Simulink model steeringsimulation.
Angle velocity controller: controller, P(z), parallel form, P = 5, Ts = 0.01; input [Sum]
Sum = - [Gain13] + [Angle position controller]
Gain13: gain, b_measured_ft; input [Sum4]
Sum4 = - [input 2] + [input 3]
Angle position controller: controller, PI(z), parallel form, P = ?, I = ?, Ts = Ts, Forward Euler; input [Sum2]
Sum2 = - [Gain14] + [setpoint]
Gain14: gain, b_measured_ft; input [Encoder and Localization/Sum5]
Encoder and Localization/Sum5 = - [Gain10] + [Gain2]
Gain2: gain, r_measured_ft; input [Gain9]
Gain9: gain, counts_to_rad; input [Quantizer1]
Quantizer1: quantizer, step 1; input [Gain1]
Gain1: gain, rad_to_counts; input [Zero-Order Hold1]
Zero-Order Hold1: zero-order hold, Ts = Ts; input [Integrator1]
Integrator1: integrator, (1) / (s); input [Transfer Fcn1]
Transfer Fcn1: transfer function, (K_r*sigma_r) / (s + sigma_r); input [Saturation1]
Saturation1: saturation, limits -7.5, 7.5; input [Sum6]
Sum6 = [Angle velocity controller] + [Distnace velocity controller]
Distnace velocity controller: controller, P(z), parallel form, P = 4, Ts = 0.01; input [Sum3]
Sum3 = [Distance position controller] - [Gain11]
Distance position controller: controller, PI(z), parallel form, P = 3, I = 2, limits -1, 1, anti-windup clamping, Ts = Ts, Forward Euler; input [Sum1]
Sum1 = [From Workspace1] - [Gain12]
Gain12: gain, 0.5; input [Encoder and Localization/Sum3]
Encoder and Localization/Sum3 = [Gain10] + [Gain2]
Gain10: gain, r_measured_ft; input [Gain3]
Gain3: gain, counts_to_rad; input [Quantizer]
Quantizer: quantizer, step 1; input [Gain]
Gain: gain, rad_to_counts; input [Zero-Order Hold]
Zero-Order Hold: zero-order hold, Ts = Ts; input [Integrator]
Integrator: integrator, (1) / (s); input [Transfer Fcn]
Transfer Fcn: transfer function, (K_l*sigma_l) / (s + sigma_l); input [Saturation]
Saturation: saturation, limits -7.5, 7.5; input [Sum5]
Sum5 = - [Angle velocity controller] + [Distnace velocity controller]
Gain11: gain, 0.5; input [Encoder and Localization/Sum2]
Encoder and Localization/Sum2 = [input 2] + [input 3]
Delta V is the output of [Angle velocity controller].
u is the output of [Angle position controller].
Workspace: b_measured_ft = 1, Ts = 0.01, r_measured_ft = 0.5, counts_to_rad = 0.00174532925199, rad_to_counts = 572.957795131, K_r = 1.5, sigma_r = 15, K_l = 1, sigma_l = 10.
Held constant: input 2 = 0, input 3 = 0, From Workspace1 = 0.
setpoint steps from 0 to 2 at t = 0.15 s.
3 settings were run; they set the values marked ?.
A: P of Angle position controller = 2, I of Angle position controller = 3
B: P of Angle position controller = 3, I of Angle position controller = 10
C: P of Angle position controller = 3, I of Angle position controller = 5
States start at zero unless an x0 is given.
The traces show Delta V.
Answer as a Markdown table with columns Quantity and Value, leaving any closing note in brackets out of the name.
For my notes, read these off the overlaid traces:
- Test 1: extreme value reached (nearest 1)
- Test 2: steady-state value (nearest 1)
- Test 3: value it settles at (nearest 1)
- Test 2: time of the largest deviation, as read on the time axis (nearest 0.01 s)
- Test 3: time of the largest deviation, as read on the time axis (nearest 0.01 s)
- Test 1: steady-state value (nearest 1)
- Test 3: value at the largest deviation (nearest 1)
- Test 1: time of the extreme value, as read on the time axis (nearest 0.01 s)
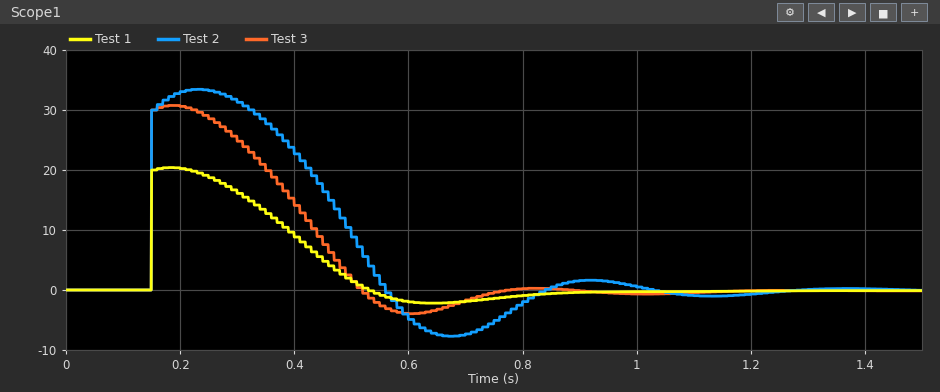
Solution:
| Quantity | Value |
|---|---|
| Test 1: extreme value reached | 20 |
| Test 2: steady-state value | 0 |
| Test 3: value it settles at | 0 |
| Test 2: time of the largest deviation, as read on the time axis | 0.23 s |
| Test 3: time of the largest deviation, as read on the time axis | 0.18 s |
| Test 1: steady-state value | 0 |
| Test 3: value at the largest deviation | 31 |
| Test 1: time of the extreme value, as read on the time axis | 0.18 s |
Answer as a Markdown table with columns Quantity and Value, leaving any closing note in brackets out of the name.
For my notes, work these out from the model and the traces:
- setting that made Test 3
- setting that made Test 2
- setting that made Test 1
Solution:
| Quantity | Value |
|---|---|
| setting that made Test 3 | C |
| setting that made Test 2 | B |
| setting that made Test 1 | A |
